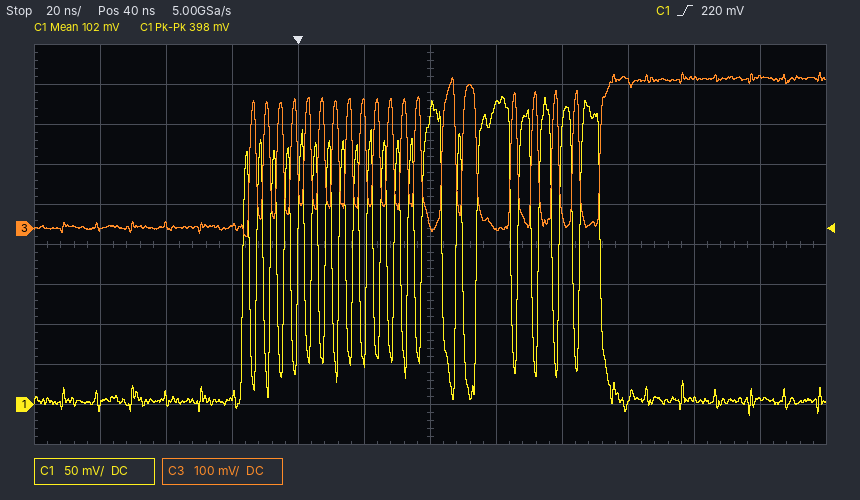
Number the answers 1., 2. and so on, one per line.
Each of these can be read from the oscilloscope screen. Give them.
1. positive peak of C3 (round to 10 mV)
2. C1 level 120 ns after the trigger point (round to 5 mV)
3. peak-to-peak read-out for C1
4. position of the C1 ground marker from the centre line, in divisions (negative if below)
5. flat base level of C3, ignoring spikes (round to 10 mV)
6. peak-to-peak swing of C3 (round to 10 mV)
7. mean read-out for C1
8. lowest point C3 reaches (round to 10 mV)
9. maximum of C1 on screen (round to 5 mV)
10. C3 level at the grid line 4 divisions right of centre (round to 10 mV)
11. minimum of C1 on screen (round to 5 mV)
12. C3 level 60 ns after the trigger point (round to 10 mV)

1. 390 mV
2. 5 mV
3. 398 mV
4. -4.0 div
5. 0 mV
6. 410 mV
7. 102 mV
8. -20 mV
9. 385 mV
10. 380 mV
11. -15 mV
12. 0 mV
